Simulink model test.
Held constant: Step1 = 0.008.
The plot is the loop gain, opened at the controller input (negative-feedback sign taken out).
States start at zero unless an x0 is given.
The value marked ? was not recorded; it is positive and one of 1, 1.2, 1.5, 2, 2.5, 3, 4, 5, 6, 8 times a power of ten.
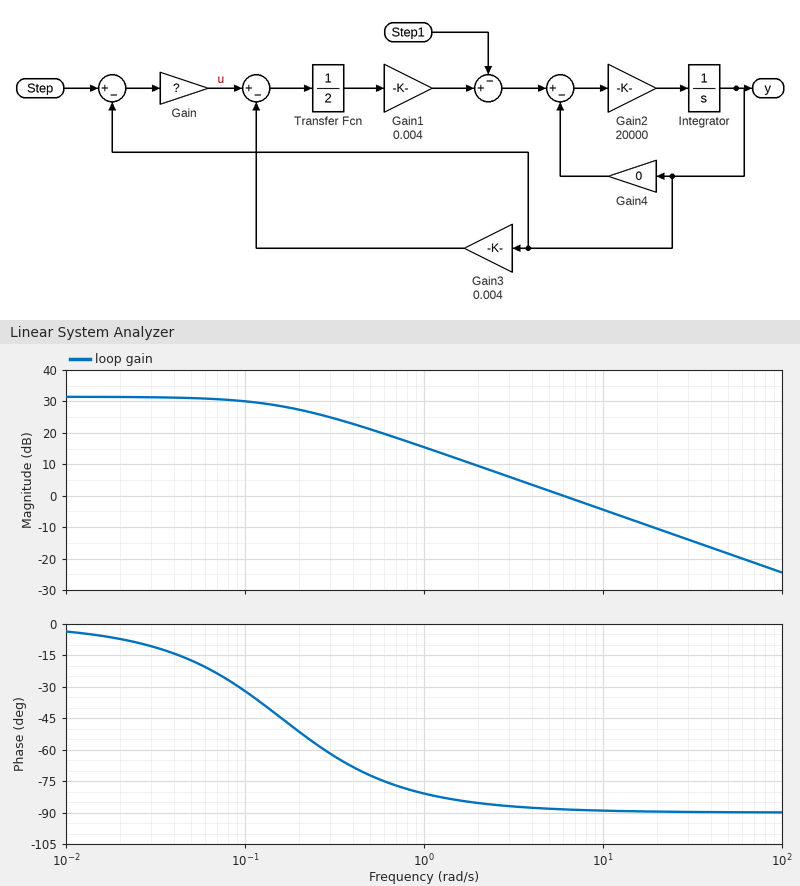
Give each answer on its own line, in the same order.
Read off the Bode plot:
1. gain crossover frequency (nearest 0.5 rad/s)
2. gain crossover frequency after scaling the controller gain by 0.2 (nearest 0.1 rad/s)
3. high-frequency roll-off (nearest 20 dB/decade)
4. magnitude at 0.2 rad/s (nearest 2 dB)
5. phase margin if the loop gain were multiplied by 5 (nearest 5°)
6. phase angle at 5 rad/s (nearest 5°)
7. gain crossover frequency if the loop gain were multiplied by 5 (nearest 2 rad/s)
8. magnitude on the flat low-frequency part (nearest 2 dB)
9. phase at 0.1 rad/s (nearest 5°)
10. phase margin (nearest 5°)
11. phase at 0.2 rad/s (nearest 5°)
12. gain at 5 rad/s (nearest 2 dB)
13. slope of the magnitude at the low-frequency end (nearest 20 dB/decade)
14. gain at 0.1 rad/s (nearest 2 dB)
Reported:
6.0 rad/s
1.2 rad/s
-20 dB/decade
28 dB
90°
-90°
30 rad/s
32 dB
-30°
90°
-50°
2 dB
0 dB/decade
30 dB
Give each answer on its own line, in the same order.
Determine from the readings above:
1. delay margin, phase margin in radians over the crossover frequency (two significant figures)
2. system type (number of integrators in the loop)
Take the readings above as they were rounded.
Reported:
0.26 s
0
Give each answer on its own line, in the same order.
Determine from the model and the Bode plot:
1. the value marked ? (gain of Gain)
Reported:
0.15
